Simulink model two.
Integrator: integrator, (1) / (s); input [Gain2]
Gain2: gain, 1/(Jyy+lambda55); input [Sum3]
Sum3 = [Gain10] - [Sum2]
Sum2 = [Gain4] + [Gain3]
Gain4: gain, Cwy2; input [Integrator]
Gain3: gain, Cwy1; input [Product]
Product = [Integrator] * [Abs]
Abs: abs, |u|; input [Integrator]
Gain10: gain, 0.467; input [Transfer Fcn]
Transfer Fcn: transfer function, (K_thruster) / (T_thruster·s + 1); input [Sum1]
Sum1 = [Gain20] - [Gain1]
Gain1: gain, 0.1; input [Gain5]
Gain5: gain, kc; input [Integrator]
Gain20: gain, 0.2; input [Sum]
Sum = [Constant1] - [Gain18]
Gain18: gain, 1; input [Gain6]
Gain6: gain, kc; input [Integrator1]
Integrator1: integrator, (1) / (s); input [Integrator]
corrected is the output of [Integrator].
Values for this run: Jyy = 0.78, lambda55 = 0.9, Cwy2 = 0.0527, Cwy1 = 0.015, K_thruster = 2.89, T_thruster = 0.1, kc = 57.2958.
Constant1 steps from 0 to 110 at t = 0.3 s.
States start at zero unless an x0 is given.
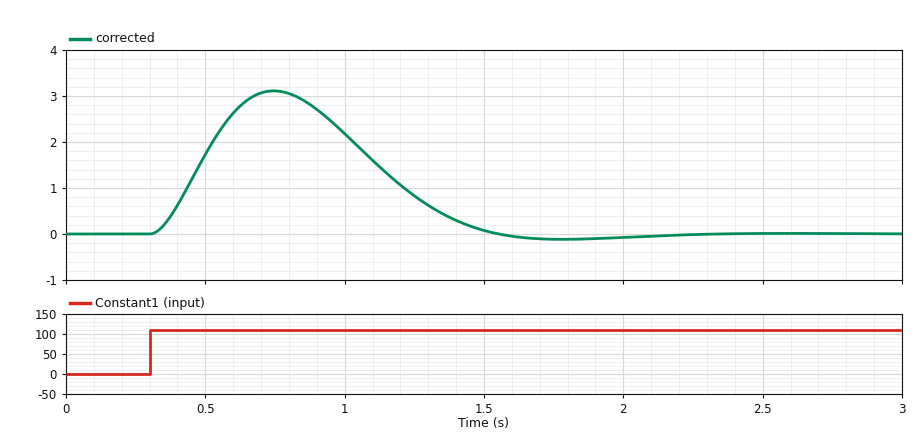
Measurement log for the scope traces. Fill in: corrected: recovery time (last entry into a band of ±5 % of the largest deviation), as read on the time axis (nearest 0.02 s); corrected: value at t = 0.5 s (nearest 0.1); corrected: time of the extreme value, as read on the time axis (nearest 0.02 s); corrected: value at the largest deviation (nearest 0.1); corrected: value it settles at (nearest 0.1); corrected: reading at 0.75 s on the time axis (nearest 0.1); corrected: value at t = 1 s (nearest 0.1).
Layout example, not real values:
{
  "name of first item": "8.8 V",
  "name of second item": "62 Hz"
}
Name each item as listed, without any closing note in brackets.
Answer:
{
  "corrected: recovery time (last entry into a band of ±5 % of the largest deviation), as read on the time axis": "1.46 s",
  "corrected: value at t = 0.5 s": "1.7",
  "corrected: time of the extreme value, as read on the time axis": "0.74 s",
  "corrected: value at the largest deviation": "3.1",
  "corrected: value it settles at": "0.0",
  "corrected: reading at 0.75 s on the time axis": "3.1",
  "corrected: value at t = 1 s": "2.2"
}
